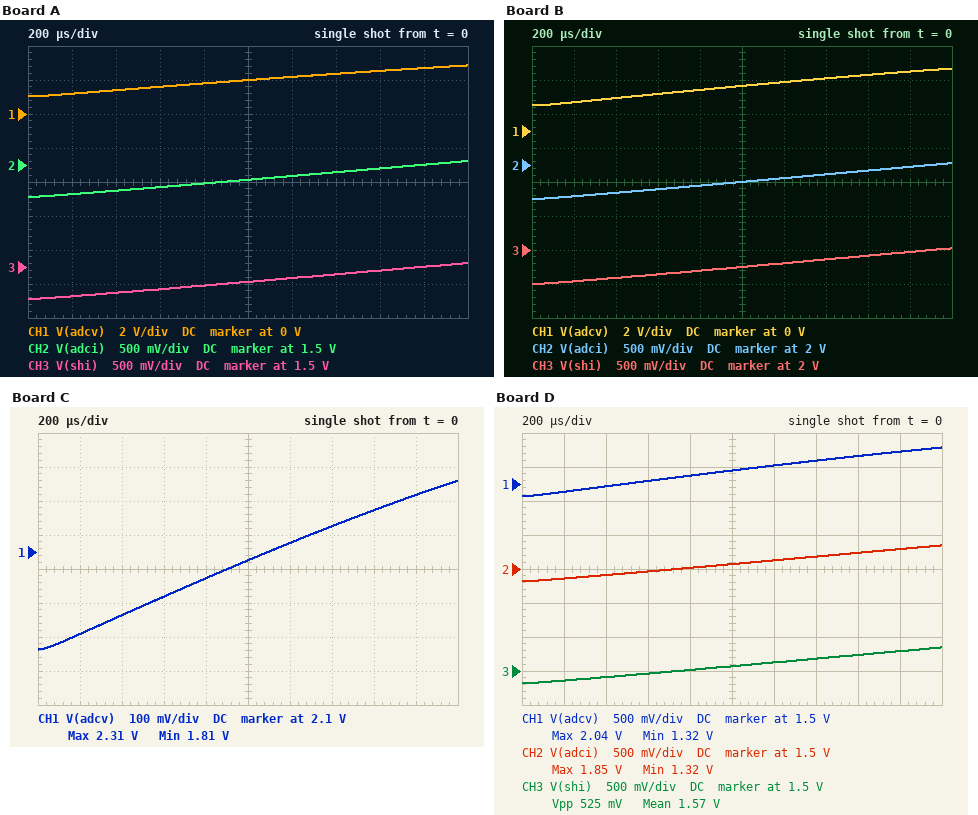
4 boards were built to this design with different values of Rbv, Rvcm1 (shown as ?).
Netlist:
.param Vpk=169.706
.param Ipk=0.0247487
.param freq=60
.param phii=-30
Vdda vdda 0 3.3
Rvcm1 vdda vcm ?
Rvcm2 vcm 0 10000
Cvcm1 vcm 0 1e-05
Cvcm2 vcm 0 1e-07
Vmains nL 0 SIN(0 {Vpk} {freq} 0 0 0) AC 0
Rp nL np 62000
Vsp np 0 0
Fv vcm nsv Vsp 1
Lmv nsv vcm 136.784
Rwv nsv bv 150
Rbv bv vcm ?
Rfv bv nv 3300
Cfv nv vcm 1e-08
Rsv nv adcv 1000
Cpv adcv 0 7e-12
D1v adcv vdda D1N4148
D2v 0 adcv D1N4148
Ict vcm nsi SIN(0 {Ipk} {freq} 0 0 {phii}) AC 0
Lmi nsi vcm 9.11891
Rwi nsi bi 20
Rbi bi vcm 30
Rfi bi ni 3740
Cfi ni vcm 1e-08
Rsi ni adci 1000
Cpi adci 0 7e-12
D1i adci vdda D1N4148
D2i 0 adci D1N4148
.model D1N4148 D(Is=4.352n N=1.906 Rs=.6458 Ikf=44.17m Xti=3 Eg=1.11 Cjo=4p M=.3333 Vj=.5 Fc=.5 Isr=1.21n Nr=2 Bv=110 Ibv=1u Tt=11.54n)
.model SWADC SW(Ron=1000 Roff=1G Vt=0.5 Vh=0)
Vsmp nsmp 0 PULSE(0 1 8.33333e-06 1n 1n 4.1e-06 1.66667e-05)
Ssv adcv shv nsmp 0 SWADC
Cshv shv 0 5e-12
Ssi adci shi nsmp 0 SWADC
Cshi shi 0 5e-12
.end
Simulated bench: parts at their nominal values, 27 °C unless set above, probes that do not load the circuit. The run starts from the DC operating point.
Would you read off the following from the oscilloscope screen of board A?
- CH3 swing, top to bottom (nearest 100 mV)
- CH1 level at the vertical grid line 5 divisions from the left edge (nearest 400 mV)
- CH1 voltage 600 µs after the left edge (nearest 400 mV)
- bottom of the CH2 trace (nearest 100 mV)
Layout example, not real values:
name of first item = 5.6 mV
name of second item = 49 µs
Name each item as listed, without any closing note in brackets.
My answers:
CH3 swing, top to bottom = 500 mV
CH1 level at the vertical grid line 5 divisions from the left edge = 2.0 V
CH1 voltage 600 µs after the left edge = 1.6 V
bottom of the CH2 trace = 1.0 V
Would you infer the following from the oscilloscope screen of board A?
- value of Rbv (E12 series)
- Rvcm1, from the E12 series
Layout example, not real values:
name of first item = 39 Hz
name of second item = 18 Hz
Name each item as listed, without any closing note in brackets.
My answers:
value of Rbv = 1 kΩ
Rvcm1, from the E12 series = 22 kΩ
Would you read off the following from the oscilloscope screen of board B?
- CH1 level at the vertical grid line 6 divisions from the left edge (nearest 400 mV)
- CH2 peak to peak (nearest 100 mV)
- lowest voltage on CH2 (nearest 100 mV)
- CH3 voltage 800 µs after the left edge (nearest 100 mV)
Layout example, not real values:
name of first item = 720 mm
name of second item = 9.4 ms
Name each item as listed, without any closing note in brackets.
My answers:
CH1 level at the vertical grid line 6 divisions from the left edge = 2.8 V
CH2 peak to peak = 500 mV
lowest voltage on CH2 = 1.5 V
CH3 voltage 800 µs after the left edge = 1.7 V
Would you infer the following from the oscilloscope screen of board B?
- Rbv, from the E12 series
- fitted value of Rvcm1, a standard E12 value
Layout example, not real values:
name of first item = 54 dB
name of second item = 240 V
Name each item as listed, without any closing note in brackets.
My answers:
Rbv, from the E12 series = 1.2 kΩ
fitted value of Rvcm1, a standard E12 value = 12 kΩ
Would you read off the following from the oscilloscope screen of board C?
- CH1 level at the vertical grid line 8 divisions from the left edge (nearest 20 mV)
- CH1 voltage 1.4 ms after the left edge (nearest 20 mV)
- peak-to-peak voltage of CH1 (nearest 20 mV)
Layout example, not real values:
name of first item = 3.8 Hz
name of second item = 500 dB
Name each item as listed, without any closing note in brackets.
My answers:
CH1 level at the vertical grid line 8 divisions from the left edge = 2.22 V
CH1 voltage 1.4 ms after the left edge = 2.18 V
peak-to-peak voltage of CH1 = 500 mV
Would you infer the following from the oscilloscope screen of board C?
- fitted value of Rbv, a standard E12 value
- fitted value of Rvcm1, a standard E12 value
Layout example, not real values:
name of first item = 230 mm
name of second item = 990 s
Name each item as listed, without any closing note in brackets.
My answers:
fitted value of Rbv, a standard E12 value = 270 Ω
fitted value of Rvcm1, a standard E12 value = 8.2 kΩ
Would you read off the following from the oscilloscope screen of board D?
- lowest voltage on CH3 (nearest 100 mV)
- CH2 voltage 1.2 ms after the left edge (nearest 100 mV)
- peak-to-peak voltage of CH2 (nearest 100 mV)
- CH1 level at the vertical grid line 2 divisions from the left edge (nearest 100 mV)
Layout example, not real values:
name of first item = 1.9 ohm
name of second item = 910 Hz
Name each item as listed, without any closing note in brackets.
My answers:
lowest voltage on CH3 = 1.3 V
CH2 voltage 1.2 ms after the left edge = 1.6 V
peak-to-peak voltage of CH2 = 500 mV
CH1 level at the vertical grid line 2 divisions from the left edge = 1.5 V
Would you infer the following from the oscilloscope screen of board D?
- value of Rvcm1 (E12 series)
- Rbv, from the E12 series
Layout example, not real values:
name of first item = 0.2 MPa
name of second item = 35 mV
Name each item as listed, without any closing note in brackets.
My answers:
value of Rvcm1 = 15 kΩ
Rbv, from the E12 series = 390 Ω
